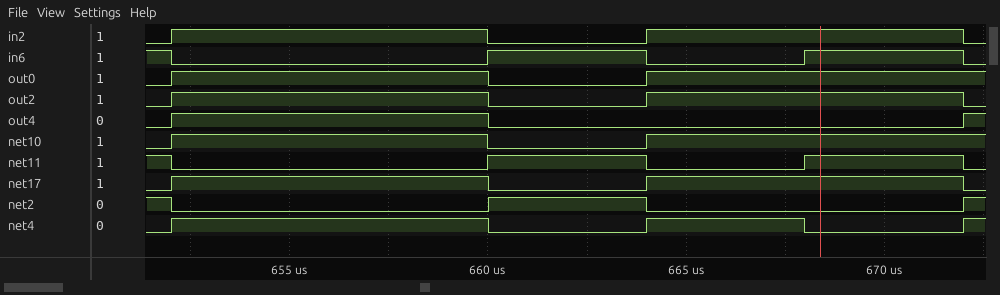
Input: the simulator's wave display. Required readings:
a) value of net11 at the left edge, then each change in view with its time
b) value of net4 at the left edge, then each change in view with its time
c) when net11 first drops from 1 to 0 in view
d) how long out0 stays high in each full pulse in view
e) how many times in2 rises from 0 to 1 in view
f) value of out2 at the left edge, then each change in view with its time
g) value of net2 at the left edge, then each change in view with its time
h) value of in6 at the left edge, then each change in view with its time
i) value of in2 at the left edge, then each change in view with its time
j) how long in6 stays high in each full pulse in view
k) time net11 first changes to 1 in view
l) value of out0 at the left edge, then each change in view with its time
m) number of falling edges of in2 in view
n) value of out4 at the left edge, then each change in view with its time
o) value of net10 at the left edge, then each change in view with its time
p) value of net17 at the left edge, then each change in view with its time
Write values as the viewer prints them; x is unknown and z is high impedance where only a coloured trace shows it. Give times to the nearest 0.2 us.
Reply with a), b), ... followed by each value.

a) 1, 0 at 652 us, 1 at 660 us, 0 at 664 us, 1 at 668 us, 0 at 672 us
b) 0, 1 at 652 us, 0 at 660 us, 1 at 664 us, 0 at 668 us, 1 at 672 us
c) 652 us
d) 8 us
e) 2
f) 0, 1 at 652 us, 0 at 660 us, 1 at 664 us, 0 at 672 us
g) 1, 0 at 652 us, 1 at 660 us, 0 at 664 us, 1 at 672 us
h) 1, 0 at 652 us, 1 at 660 us, 0 at 664 us, 1 at 668 us, 0 at 672 us
i) 0, 1 at 652 us, 0 at 660 us, 1 at 664 us, 0 at 672 us
j) 4 us, 4 us
k) 660 us
l) 0, 1 at 652 us, 0 at 660 us, 1 at 664 us
m) 2
n) 0, 1 at 652 us, 0 at 660 us, 1 at 672 us
o) 0, 1 at 652 us, 0 at 660 us, 1 at 664 us
p) 0, 1 at 652 us, 0 at 660 us, 1 at 664 us, 0 at 672 us
